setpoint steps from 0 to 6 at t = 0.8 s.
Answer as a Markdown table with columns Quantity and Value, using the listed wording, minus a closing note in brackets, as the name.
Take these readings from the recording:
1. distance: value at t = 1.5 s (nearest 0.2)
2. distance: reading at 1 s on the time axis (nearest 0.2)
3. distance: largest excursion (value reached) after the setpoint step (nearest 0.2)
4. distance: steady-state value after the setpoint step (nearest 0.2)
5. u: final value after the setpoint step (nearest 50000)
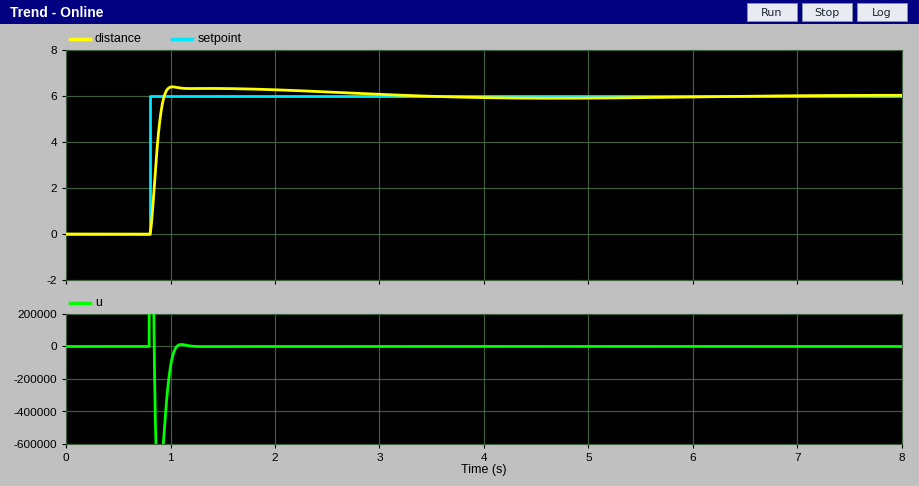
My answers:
| Quantity | Value |
|---|---|
| distance: value at t = 1.5 s | 6.4 |
| distance: reading at 1 s on the time axis | 6.4 |
| distance: largest excursion (value reached) after the setpoint step | 6.4 |
| distance: steady-state value after the setpoint step | 6.0 |
| u: final value after the setpoint step | 0 |
